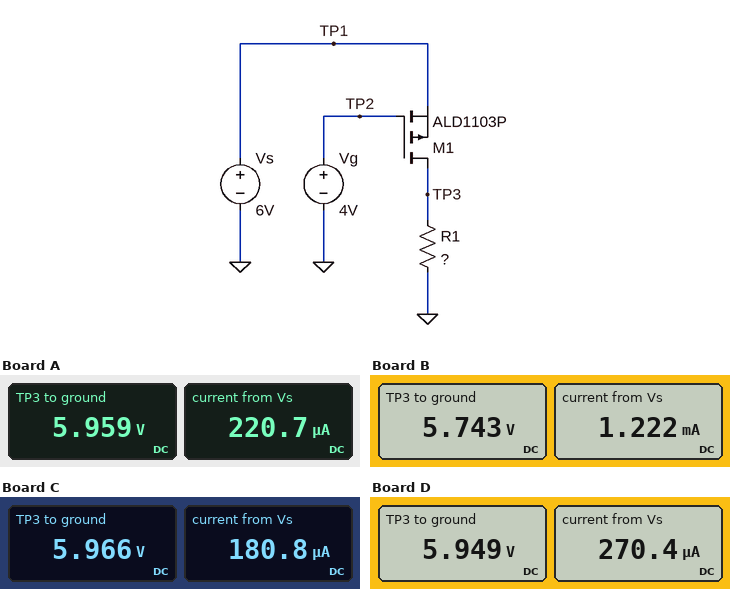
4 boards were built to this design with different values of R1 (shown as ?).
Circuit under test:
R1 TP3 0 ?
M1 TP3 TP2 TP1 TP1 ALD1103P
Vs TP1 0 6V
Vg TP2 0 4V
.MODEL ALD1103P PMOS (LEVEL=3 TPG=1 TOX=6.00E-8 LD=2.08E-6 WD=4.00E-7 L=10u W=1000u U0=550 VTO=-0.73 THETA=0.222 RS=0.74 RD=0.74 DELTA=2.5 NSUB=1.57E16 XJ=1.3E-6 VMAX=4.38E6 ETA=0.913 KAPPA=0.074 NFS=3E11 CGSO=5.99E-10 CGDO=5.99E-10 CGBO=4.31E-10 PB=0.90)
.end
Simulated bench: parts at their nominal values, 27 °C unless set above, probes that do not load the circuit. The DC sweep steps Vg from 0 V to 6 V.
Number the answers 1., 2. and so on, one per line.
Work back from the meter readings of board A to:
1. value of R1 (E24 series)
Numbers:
1. 27 kΩ
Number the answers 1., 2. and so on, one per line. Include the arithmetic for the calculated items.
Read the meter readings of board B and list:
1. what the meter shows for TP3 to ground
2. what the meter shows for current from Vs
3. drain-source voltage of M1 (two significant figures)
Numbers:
1. 5.743 V
2. 1.222 mA
3. 5.743 V - 6 V = -260 mV
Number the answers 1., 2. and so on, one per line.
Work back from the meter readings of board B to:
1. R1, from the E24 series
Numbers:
1. 4.7 kΩ
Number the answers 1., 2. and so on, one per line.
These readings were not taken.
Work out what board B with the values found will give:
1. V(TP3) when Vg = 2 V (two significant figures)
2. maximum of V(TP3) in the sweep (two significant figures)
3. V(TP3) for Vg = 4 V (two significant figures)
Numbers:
1. 5.9 V
2. 5.9 V
3. 5.7 V
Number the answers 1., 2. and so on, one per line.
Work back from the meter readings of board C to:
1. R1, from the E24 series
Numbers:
1. 33 kΩ
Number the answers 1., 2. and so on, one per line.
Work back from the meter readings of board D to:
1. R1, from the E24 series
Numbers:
1. 22 kΩ
